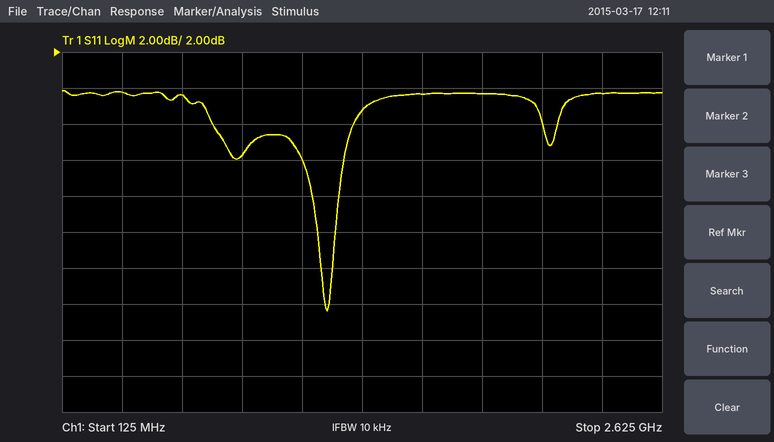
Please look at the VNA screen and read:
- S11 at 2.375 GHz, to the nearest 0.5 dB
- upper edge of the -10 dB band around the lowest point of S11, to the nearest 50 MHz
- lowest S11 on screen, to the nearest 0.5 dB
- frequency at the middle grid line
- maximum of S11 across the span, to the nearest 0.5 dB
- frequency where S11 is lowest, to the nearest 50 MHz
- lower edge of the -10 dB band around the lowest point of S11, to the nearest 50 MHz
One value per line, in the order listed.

-0.5 dB
1.25 GHz
-12.5 dB
1.375 GHz
0.0 dB
1.25 GHz
1.20 GHz
